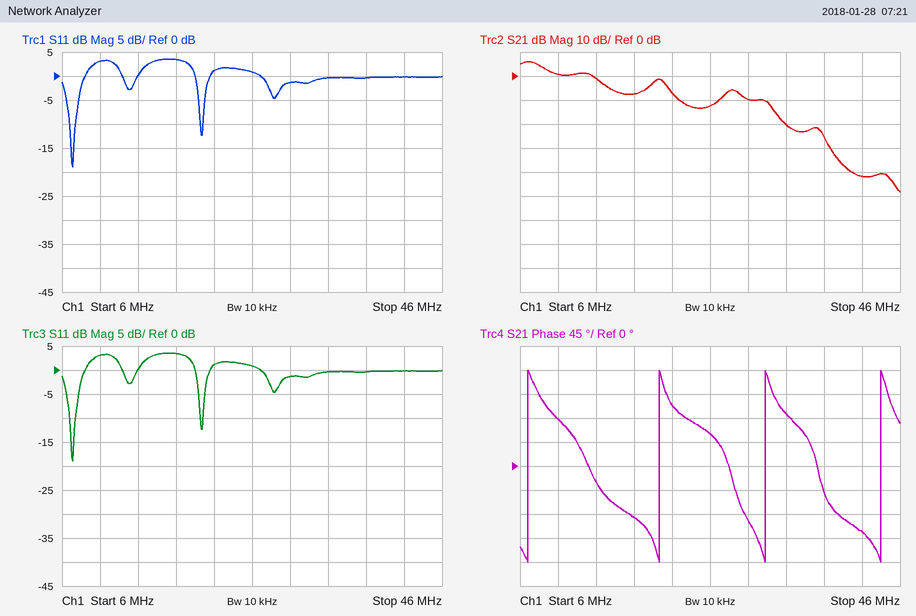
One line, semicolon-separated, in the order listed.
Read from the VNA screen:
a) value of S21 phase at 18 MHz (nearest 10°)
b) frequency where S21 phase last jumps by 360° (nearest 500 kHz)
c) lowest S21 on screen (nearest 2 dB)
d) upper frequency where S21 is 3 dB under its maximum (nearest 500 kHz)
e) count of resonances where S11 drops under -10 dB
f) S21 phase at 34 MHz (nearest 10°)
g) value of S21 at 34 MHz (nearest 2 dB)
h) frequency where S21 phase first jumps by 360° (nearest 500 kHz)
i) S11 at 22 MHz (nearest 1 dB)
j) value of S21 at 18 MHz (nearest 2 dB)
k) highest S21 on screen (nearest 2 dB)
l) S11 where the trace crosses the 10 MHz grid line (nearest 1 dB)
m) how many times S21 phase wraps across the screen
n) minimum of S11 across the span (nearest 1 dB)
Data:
-100°; 44.0 MHz; -48 dB; 8.5 MHz; 2; 100°; -20 dB; 7.0 MHz; 1 dB; -8 dB; 6 dB; 3 dB; 4; -19 dB
